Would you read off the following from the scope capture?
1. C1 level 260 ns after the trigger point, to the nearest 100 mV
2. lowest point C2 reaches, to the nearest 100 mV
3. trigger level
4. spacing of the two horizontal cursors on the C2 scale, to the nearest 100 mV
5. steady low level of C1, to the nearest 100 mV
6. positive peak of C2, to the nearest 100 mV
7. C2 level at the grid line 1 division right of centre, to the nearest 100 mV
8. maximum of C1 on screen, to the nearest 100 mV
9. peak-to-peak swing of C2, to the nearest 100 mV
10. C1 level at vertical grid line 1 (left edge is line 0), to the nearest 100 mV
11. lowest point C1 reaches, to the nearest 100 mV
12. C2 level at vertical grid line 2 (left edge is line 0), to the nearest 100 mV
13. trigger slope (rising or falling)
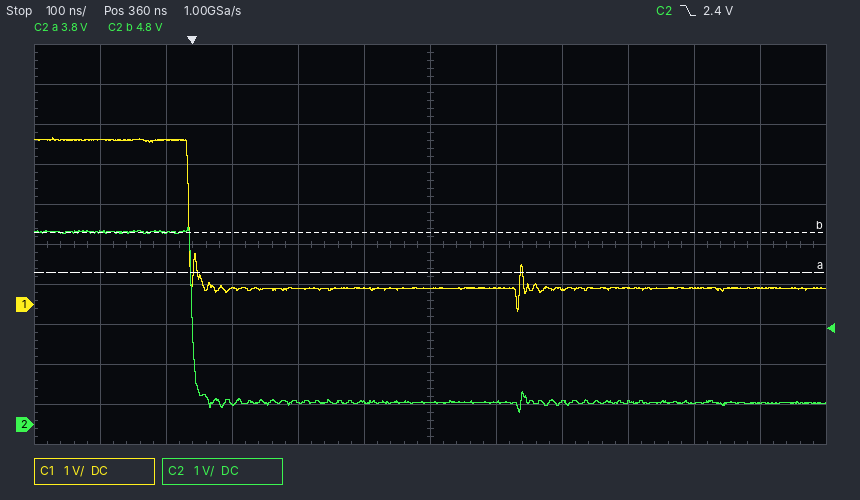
400 mV
300 mV
2.4 V
1.0 V
400 mV
4.9 V
600 mV
4.2 V
4.6 V
4.1 V
-200 mV
4.8 V
falling
